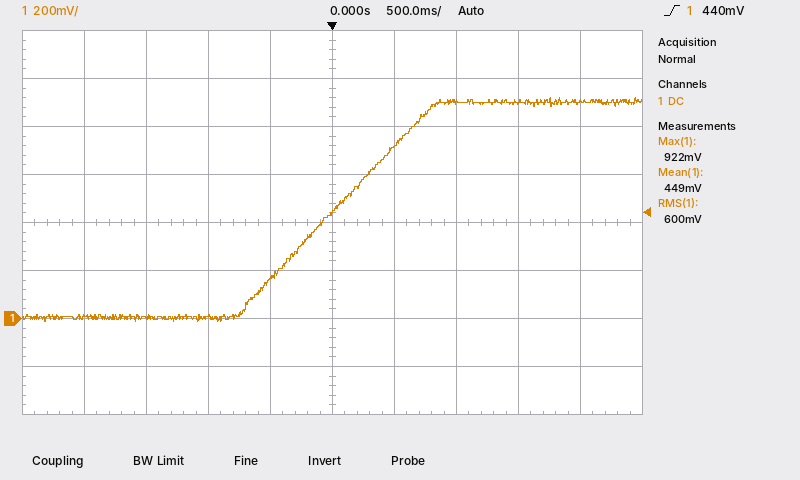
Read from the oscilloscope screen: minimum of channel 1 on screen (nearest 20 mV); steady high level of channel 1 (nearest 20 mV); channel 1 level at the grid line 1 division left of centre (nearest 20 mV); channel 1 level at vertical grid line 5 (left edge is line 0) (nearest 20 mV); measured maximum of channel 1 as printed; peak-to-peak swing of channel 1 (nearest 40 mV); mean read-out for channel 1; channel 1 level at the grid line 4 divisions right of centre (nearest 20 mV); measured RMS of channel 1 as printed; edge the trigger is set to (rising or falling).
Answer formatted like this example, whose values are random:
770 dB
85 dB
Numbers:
-20 mV
900 mV
160 mV
440 mV
922 mV
920 mV
449 mV
900 mV
600 mV
rising
